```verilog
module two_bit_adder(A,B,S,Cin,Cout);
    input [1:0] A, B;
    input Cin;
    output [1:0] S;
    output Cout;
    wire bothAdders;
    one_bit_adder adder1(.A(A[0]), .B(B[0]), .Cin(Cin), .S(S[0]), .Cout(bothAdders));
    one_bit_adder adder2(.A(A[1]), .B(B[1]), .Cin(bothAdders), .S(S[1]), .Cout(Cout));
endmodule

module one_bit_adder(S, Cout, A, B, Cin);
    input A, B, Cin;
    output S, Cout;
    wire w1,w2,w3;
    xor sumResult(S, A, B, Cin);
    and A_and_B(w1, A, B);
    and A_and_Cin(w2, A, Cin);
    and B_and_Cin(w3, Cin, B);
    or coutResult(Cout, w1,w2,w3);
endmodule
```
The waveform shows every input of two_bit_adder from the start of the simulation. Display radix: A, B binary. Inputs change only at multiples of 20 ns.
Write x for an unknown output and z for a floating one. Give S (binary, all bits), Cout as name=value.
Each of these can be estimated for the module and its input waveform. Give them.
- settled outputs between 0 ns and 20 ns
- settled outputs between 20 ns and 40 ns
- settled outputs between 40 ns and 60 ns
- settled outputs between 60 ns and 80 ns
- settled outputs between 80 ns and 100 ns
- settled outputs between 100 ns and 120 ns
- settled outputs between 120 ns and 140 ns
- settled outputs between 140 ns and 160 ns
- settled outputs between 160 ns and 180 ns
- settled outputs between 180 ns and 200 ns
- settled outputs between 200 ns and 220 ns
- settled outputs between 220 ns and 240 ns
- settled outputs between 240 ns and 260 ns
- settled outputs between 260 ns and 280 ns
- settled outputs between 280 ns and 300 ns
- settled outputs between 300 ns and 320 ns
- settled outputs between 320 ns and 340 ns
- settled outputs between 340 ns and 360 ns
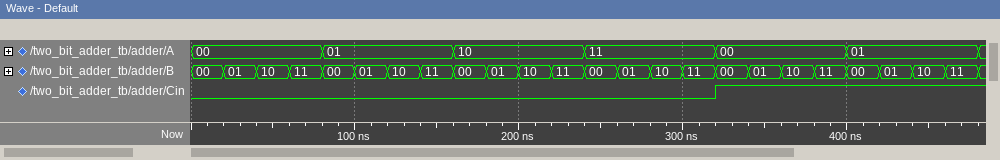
S=00, Cout=0
S=01, Cout=0
S=10, Cout=0
S=11, Cout=0
S=01, Cout=0
S=10, Cout=0
S=11, Cout=0
S=00, Cout=1
S=10, Cout=0
S=11, Cout=0
S=00, Cout=1
S=01, Cout=1
S=11, Cout=0
S=00, Cout=1
S=01, Cout=1
S=10, Cout=1
S=01, Cout=0
S=10, Cout=0
